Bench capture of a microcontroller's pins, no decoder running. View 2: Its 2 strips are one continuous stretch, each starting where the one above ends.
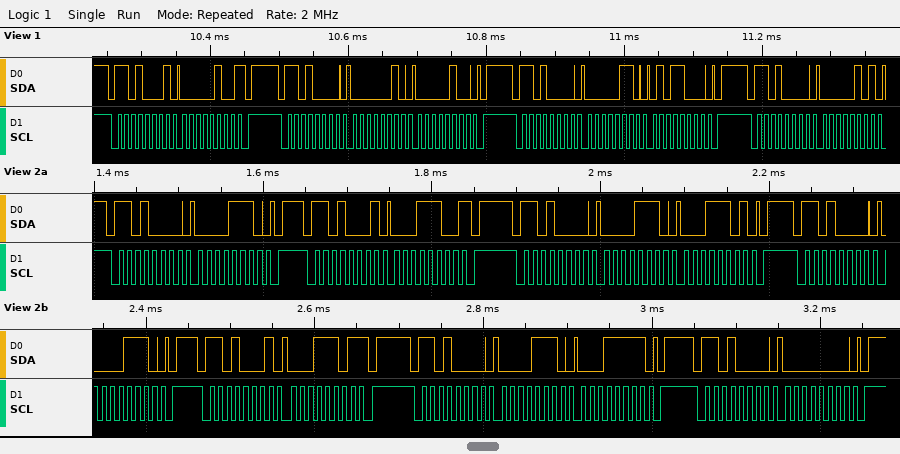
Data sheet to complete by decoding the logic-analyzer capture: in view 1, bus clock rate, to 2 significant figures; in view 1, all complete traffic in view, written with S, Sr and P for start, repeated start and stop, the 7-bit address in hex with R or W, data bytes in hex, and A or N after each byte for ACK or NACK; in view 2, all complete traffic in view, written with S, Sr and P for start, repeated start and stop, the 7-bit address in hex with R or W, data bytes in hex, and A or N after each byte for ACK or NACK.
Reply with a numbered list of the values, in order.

1. 100 kHz
2. S 68R A 04 N P S 68W A 02 A 04 A P S 68W A 06 A 58 A P S 68W A 05 A
3. S 68W A 0E A P S 68R A 1C N P S 68W A 0E A 1D A P S 68W A 0E A P S 68R A 1D N P S 68W A 0E A 1F A P S 68W A 00 A P
